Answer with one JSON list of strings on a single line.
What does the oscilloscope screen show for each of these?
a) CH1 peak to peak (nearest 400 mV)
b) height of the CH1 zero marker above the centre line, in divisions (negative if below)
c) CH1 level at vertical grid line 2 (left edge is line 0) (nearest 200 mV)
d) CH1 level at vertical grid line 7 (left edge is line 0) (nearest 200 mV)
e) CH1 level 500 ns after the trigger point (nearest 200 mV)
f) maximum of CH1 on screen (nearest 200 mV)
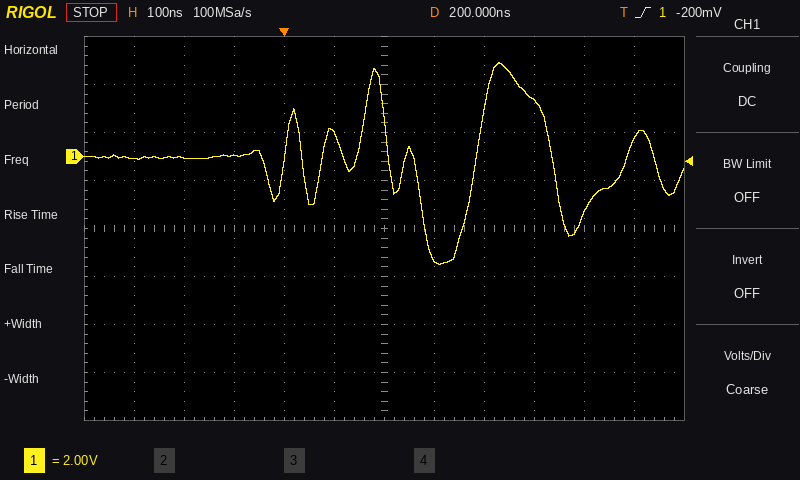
["8.4 V", "+1.5 div", "0.0 V", "-4.2 V", "2.4 V", "4.0 V"]
